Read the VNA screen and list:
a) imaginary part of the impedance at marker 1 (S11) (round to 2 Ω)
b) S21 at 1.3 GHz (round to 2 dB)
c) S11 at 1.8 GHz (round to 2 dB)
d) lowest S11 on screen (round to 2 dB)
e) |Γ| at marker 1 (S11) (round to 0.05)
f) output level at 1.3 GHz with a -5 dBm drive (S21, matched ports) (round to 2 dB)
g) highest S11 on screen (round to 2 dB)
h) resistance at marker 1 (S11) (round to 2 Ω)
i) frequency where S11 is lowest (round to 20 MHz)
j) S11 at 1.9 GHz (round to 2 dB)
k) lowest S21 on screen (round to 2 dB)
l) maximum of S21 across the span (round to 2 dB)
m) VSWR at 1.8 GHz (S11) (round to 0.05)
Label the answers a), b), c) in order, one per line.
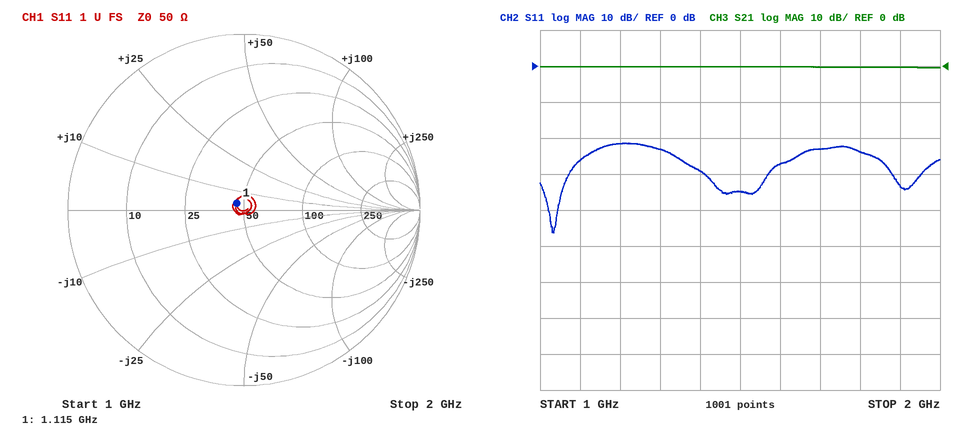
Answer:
a) +4 Ω
b) 0 dB
c) -24 dB
d) -46 dB
e) 0.05
f) -6 dBm
g) -22 dB
h) 46 Ω
i) 1.04 GHz
j) -34 dB
k) 0 dB
l) 0 dB
m) 1.15
